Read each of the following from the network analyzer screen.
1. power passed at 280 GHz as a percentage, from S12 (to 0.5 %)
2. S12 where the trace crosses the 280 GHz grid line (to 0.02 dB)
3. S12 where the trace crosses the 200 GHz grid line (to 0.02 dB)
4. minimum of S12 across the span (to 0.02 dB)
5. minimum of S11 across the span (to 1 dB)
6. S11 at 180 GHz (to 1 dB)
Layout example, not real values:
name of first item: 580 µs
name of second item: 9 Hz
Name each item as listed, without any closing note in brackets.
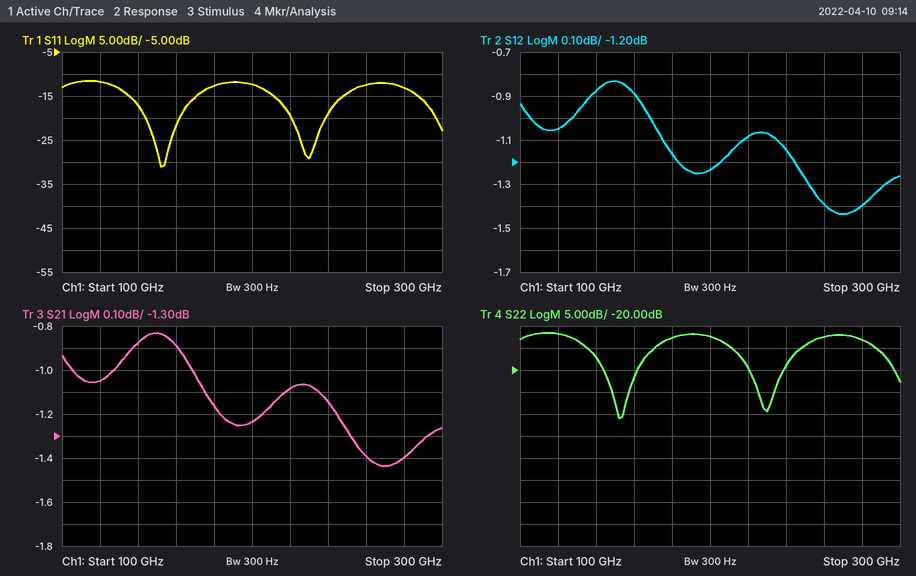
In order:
power passed at 280 GHz as a percentage, from S12: 72.5 %
S12 where the trace crosses the 280 GHz grid line: -1.40 dB
S12 where the trace crosses the 200 GHz grid line: -1.24 dB
minimum of S12 across the span: -1.44 dB
minimum of S11 across the span: -31 dB
S11 at 180 GHz: -13 dB
